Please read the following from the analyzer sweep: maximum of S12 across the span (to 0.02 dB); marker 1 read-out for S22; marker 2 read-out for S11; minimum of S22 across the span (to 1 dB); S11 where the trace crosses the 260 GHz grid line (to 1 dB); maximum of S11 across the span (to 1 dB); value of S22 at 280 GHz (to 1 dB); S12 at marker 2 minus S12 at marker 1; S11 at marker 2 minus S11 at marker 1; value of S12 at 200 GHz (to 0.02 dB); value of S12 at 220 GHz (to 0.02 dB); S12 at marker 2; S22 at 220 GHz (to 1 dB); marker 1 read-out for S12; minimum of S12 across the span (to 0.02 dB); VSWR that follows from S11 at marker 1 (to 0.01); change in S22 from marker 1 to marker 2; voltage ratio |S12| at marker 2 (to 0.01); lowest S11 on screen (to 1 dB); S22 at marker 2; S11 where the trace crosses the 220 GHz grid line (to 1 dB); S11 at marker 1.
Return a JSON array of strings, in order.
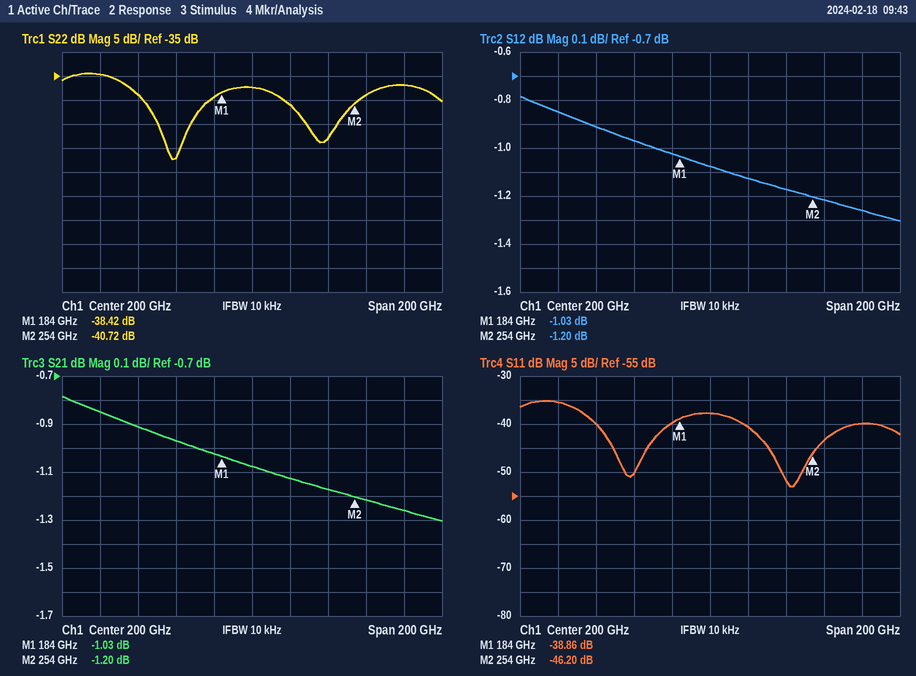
["-0.78 dB", "-38.42 dB", "-46.20 dB", "-52 dB", "-43 dB", "-35 dB", "-37 dB", "-0.17 dB", "-7.34 dB", "-1.08 dB", "-1.12 dB", "-1.20 dB", "-41 dB", "-1.03 dB", "-1.30 dB", "1.02", "-2.30 dB", "0.87", "-53 dB", "-40.72 dB", "-41 dB", "-38.86 dB"]
